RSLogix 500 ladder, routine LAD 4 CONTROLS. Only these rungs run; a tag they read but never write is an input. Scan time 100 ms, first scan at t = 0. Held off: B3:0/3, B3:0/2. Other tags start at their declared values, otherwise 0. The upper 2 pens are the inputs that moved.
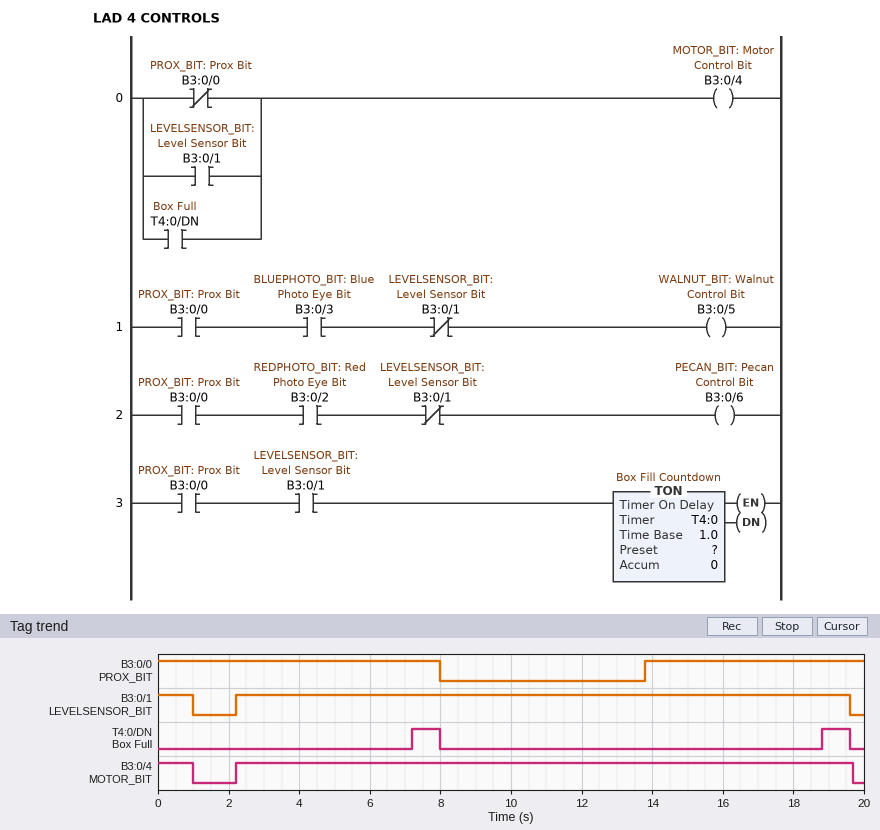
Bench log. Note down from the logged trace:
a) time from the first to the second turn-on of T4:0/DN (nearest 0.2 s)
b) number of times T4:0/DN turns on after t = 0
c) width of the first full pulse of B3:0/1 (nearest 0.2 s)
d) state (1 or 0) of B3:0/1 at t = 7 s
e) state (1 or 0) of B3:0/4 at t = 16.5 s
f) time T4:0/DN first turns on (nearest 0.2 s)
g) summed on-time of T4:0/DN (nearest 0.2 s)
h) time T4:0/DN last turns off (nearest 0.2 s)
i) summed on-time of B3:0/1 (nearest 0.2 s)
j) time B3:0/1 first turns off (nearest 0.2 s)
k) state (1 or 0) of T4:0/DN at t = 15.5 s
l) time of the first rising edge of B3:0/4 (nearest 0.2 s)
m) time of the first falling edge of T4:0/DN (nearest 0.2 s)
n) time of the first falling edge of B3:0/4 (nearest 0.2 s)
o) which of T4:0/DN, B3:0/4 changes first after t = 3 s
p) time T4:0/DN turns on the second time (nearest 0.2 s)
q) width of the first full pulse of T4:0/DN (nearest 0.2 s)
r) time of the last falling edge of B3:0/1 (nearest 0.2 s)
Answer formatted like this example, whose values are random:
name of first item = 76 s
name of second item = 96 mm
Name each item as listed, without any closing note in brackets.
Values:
time from the first to the second turn-on of T4:0/DN = 11.6 s
number of times T4:0/DN turns on after t = 0 = 2
width of the first full pulse of B3:0/1 = 17.4 s
state (1 or 0) of B3:0/1 at t = 7 s = 1
state (1 or 0) of B3:0/4 at t = 16.5 s = 1
time T4:0/DN first turns on = 7.2 s
summed on-time of T4:0/DN = 1.6 s
time T4:0/DN last turns off = 19.6 s
summed on-time of B3:0/1 = 18.4 s
time B3:0/1 first turns off = 1.0 s
state (1 or 0) of T4:0/DN at t = 15.5 s = 0
time of the first rising edge of B3:0/4 = 2.2 s
time of the first falling edge of T4:0/DN = 8.0 s
time of the first falling edge of B3:0/4 = 1.0 s
which of T4:0/DN, B3:0/4 changes first after t = 3 s = T4:0/DN
time T4:0/DN turns on the second time = 18.8 s
width of the first full pulse of T4:0/DN = 0.8 s
time of the last falling edge of B3:0/1 = 19.6 s
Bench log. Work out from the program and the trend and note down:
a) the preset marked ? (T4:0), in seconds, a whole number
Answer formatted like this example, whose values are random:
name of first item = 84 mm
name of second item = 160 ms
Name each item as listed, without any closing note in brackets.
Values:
the preset marked ? (T4:0), in seconds, a whole number = 5 s
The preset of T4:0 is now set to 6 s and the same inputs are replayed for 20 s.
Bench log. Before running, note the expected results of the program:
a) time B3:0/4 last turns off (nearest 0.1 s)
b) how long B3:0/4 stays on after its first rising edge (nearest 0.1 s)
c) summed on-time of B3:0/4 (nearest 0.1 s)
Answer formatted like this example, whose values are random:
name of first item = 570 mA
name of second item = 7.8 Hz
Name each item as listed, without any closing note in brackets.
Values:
time B3:0/4 last turns off = 19.6 s
how long B3:0/4 stays on after its first rising edge = 17.4 s
summed on-time of B3:0/4 = 18.4 s
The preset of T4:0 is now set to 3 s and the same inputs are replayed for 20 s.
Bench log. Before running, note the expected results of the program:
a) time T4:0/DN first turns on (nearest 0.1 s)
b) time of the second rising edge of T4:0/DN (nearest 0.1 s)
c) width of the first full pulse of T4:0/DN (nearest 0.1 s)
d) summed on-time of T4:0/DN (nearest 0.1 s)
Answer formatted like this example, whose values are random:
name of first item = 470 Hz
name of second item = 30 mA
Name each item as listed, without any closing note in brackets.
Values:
time T4:0/DN first turns on = 5.2 s
time of the second rising edge of T4:0/DN = 16.8 s
width of the first full pulse of T4:0/DN = 2.8 s
summed on-time of T4:0/DN = 5.6 s
